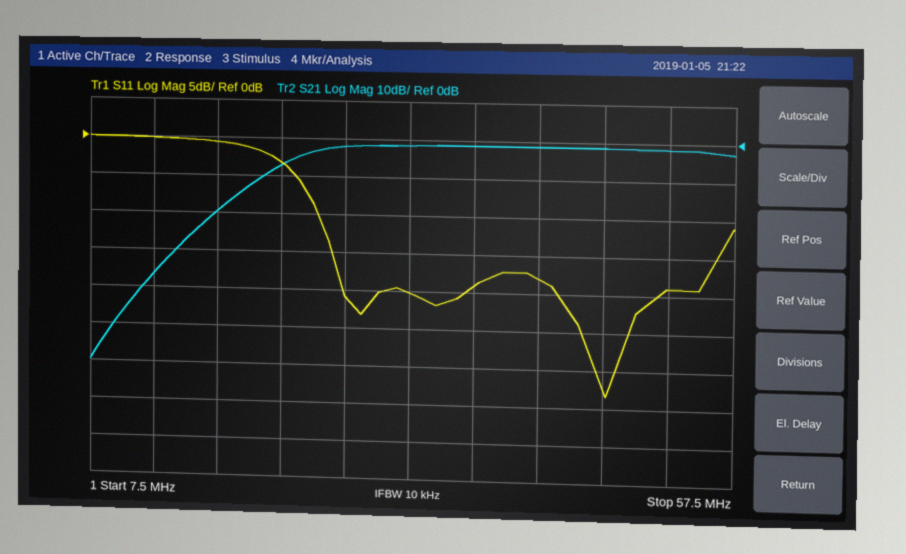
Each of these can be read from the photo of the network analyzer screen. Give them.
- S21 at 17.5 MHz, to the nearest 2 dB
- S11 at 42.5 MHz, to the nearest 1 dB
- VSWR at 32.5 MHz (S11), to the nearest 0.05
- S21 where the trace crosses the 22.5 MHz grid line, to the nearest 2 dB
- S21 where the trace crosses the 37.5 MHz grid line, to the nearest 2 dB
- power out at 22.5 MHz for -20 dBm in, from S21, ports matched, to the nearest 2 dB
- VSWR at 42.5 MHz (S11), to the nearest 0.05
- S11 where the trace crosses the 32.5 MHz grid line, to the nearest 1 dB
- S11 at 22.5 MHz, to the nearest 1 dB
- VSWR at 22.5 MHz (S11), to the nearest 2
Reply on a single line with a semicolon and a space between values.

-20 dB; -18 dB; 1.20; -8 dB; -2 dB; -28 dBm; 1.30; -20 dB; -3 dB; 6
